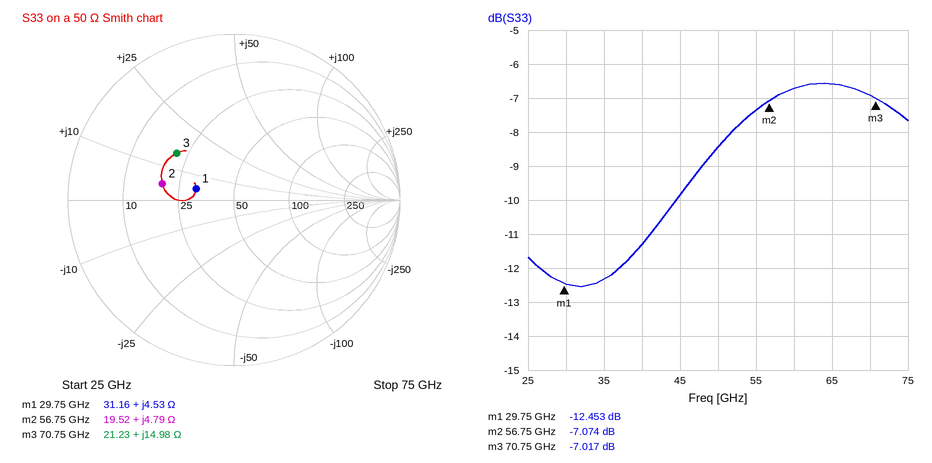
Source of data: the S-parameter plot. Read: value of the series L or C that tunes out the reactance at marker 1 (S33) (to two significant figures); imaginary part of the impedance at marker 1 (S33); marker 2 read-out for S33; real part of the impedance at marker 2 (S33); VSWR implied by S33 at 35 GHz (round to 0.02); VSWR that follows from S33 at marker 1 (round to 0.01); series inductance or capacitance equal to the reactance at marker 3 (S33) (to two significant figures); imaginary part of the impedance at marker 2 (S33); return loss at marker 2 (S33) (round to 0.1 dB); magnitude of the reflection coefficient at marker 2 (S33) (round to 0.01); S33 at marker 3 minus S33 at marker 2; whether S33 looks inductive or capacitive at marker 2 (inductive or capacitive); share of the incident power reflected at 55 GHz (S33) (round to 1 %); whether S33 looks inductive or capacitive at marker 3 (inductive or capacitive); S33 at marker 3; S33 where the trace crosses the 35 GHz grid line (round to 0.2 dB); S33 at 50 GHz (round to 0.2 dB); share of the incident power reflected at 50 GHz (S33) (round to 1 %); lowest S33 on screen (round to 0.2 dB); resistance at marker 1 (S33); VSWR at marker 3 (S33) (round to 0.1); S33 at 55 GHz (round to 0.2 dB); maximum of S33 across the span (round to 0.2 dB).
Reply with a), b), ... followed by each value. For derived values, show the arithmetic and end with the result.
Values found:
a) C = 1/(2π × 29.75 GHz × 4.53 Ω) ≈ 1.2 pF
b) +4.53 Ω
c) -7.074 dB
d) 19.52 Ω
e) |Γ| = 10^(-12.4/20) = 0.2399; VSWR = (1 + 0.2399)/(1 − 0.2399) ≈ 1.63, so 1.64 to the nearest 0.02
f) (1 + 0.2384)/(1 − 0.2384) ≈ 1.63
g) L = 14.98 Ω/(2π × 70.75 GHz) ≈ 34 pH
h) +4.79 Ω
i) 7.1 dB
j) 10^(-7.074/20) ≈ 0.44
k) -7.017 − (-7.074) = 0.057 dB
l) inductive
m) 10^(-7.4/10) ≈ 18 %
n) inductive
o) -7.017 dB
p) -12.4 dB
q) -8.4 dB
r) 10^(-8.4/10) ≈ 14 %
s) -12.6 dB
t) 31.16 Ω
u) 2.6
v) -7.4 dB
w) -6.6 dB
